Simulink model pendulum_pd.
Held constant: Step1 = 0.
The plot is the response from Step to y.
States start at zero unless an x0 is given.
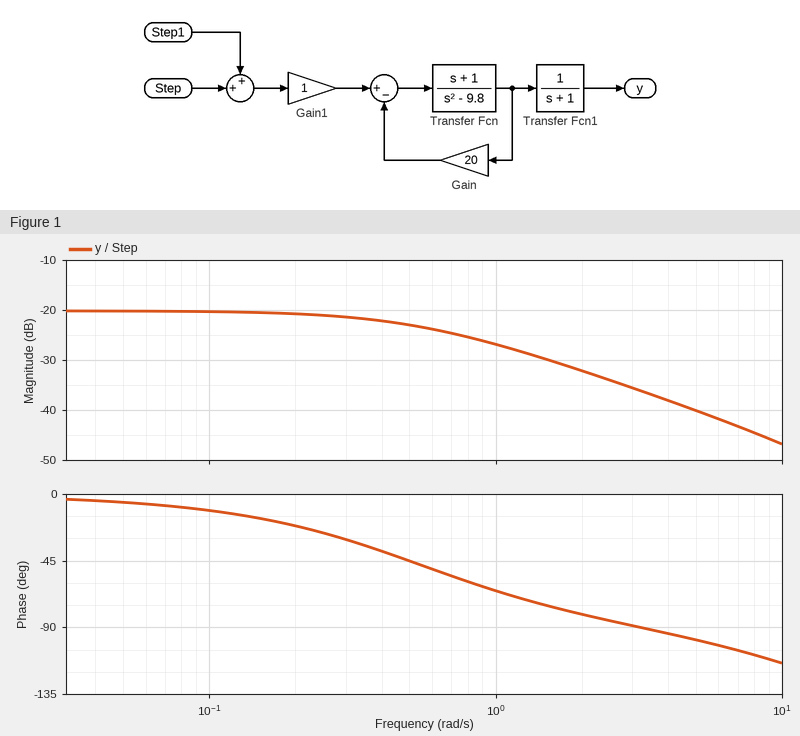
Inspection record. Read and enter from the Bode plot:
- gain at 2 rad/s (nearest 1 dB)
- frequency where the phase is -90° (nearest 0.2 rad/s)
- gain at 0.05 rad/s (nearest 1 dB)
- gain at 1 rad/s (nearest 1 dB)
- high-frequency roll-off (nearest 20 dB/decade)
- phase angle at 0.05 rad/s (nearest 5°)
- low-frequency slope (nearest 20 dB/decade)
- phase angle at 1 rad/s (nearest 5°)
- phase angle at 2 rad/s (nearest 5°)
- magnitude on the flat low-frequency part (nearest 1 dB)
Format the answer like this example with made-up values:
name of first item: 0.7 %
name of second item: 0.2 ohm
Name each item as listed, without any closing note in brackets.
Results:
gain at 2 rad/s: -32 dB
frequency where the phase is -90°: 3.2 rad/s
gain at 0.05 rad/s: -20 dB
gain at 1 rad/s: -27 dB
high-frequency roll-off: -20 dB/decade
phase angle at 0.05 rad/s: -5°
low-frequency slope: 0 dB/decade
phase angle at 1 rad/s: -65°
phase angle at 2 rad/s: -80°
magnitude on the flat low-frequency part: -20 dB
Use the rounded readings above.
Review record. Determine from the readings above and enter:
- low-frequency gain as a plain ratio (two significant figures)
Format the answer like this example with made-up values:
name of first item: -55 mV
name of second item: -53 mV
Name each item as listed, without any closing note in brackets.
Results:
low-frequency gain as a plain ratio: 0.10
